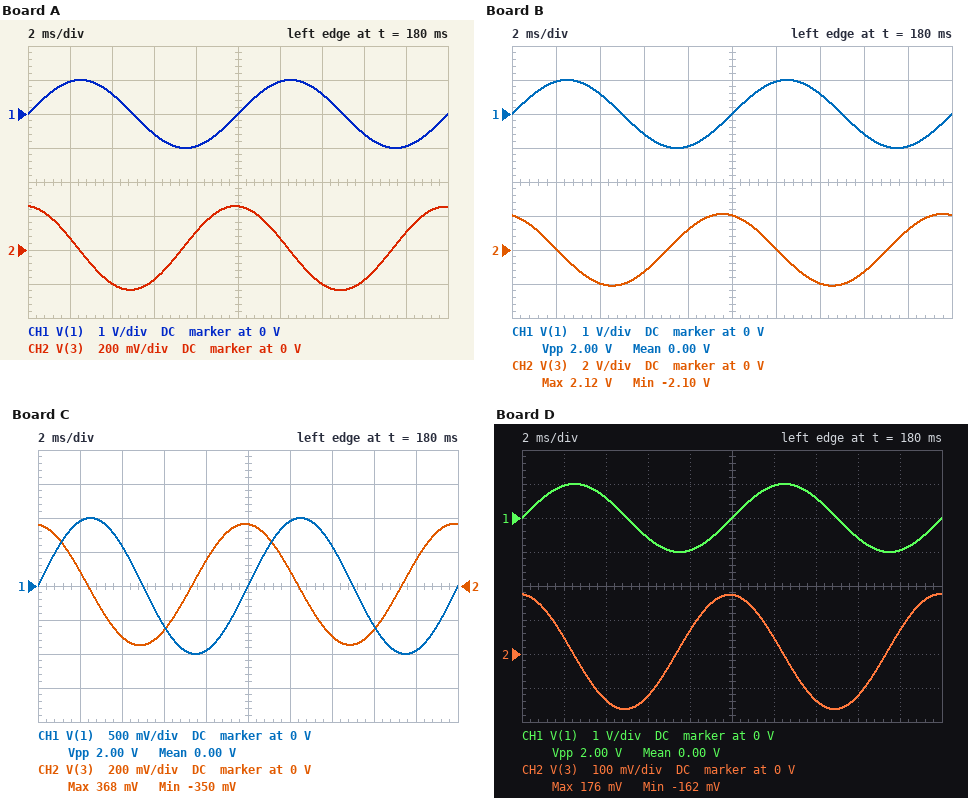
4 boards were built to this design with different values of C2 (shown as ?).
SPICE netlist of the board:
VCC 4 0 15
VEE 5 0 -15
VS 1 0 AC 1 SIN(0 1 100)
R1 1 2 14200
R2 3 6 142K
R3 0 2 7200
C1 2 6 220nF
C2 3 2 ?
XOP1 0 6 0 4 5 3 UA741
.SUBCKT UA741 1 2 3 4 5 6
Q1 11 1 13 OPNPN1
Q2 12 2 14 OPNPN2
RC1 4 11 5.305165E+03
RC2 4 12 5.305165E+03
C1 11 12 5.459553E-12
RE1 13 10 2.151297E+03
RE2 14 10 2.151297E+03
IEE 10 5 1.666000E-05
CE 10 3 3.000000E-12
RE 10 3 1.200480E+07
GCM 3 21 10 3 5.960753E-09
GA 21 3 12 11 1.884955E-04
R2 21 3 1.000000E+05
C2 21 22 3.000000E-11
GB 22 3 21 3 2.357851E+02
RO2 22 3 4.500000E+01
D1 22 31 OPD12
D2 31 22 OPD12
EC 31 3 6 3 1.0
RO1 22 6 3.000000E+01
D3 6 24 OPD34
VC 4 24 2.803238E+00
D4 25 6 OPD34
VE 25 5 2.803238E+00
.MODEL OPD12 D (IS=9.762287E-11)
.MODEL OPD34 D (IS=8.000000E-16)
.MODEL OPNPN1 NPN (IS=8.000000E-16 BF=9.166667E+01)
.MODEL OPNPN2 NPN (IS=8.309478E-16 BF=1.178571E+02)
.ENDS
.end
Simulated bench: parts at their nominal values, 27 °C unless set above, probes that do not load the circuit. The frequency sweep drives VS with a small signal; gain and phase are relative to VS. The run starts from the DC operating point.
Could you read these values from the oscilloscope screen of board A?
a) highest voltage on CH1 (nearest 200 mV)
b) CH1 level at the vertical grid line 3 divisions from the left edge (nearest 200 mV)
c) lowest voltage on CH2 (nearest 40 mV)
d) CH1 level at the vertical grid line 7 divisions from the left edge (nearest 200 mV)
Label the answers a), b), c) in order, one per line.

a) 1.0 V
b) -600 mV
c) -240 mV
d) 600 mV
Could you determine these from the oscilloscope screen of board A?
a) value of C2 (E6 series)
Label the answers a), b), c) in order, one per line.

a) 470 nF
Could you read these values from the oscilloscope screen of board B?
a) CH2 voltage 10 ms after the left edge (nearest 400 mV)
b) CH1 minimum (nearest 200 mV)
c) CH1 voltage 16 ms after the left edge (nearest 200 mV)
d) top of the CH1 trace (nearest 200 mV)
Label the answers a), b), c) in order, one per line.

a) 2.0 V
b) -1.0 V
c) -600 mV
d) 1.0 V
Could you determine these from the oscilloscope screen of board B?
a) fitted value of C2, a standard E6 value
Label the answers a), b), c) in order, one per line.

a) 68 nF
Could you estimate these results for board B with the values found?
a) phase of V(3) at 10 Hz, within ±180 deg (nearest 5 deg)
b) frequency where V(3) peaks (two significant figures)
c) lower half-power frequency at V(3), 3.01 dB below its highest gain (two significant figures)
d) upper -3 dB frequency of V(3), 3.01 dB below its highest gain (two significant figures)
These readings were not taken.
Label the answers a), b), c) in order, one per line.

a) -95 deg
b) 50 Hz
c) 40 Hz
d) 62 Hz
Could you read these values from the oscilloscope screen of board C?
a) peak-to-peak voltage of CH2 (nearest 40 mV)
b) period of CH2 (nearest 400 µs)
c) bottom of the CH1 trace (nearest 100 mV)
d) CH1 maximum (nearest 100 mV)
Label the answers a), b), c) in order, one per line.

a) 720 mV
b) 10.0 ms
c) -1.0 V
d) 1.0 V
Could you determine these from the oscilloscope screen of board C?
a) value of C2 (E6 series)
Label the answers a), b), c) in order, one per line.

a) 330 nF
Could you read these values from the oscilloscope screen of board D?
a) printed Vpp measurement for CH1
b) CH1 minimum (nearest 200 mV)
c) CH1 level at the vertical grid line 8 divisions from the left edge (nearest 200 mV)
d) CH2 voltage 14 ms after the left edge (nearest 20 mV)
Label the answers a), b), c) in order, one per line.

a) 2.00 V
b) -1.0 V
c) -600 mV
d) -140 mV
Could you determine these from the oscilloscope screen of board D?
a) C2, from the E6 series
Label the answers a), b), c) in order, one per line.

a) 680 nF
